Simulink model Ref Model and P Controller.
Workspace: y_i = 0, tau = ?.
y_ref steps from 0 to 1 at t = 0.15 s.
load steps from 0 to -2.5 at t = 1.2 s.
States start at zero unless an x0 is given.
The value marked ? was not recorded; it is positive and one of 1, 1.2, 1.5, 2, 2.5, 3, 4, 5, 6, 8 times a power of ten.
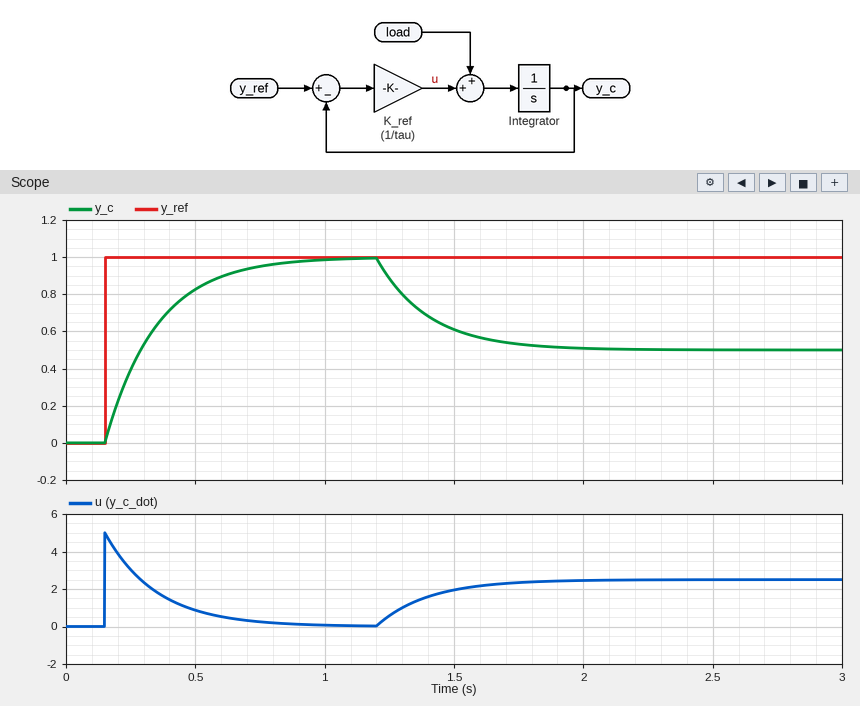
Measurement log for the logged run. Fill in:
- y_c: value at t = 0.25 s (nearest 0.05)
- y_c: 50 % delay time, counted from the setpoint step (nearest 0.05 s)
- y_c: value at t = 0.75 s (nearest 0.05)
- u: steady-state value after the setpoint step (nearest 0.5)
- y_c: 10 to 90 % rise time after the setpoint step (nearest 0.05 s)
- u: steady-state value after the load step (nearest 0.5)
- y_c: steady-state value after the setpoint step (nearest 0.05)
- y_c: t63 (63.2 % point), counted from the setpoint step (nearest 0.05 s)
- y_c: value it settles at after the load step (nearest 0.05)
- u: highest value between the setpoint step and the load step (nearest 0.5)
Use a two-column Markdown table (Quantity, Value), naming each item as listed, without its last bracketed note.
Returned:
| Quantity | Value |
|---|---|
| y_c: value at t = 0.25 s | 0.40 |
| y_c: 50 % delay time, counted from the setpoint step | 0.15 s |
| y_c: value at t = 0.75 s | 0.95 |
| u: steady-state value after the setpoint step | 0.0 |
| y_c: 10 to 90 % rise time after the setpoint step | 0.45 s |
| u: steady-state value after the load step | 2.5 |
| y_c: steady-state value after the setpoint step | 1.00 |
| y_c: t63 (63.2 % point), counted from the setpoint step | 0.20 s |
| y_c: value it settles at after the load step | 0.50 |
| u: highest value between the setpoint step and the load step | 5.0 |
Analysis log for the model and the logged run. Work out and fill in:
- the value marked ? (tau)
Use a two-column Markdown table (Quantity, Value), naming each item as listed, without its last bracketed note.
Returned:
| Quantity | Value |
|---|---|
| the value marked ? | 0.2 |
